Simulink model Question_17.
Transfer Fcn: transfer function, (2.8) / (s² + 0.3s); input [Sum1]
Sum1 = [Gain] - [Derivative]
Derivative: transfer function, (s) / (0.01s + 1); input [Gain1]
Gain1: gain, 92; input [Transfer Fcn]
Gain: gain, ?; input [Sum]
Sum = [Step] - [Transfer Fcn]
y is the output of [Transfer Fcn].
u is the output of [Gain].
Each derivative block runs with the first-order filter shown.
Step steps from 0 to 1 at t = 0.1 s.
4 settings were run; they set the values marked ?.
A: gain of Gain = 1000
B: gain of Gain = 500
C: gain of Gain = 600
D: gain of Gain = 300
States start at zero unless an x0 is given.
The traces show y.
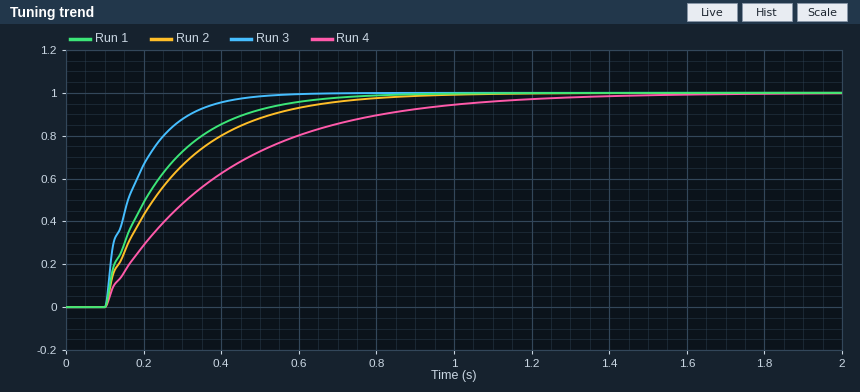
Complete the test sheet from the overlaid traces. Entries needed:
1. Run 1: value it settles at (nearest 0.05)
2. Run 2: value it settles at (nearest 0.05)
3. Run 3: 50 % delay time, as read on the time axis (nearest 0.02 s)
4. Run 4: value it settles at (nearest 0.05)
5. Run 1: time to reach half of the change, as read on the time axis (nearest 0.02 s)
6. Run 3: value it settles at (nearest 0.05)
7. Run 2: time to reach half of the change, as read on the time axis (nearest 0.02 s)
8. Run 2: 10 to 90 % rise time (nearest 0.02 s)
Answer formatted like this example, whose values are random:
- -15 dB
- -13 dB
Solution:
- 1.00
- 1.00
- 0.16 s
- 1.00
- 0.20 s
- 1.00
- 0.22 s
- 0.42 s
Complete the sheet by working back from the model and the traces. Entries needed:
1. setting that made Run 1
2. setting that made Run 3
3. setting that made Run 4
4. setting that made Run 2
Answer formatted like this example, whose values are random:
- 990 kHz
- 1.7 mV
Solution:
- C
- A
- D
- B
